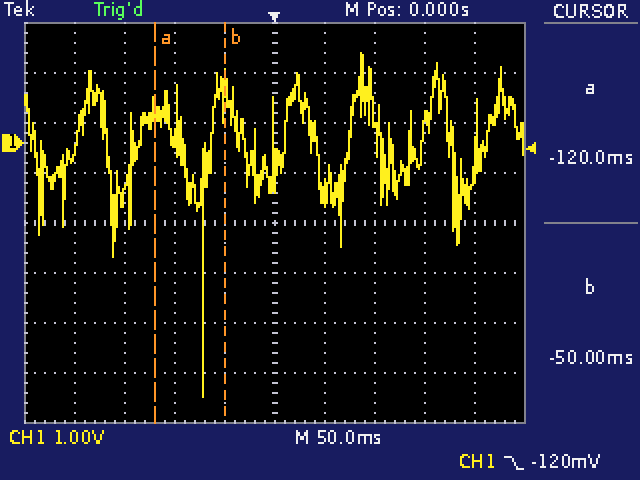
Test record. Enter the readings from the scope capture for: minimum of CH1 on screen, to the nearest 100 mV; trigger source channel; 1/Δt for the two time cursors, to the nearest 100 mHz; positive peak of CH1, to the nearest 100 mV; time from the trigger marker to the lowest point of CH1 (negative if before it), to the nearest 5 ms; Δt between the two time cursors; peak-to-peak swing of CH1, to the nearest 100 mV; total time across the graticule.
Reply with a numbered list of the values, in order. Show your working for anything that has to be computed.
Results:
1. -5.1 V
2. CH1
3. 1 / 70 ms ≈ 14.3 Hz
4. 1.8 V
5. -70 ms
6. -50 ms − (-120 ms) = 70 ms
7. 1.8 V − (-5.1 V) = 6.9 V
8. 500 ms
